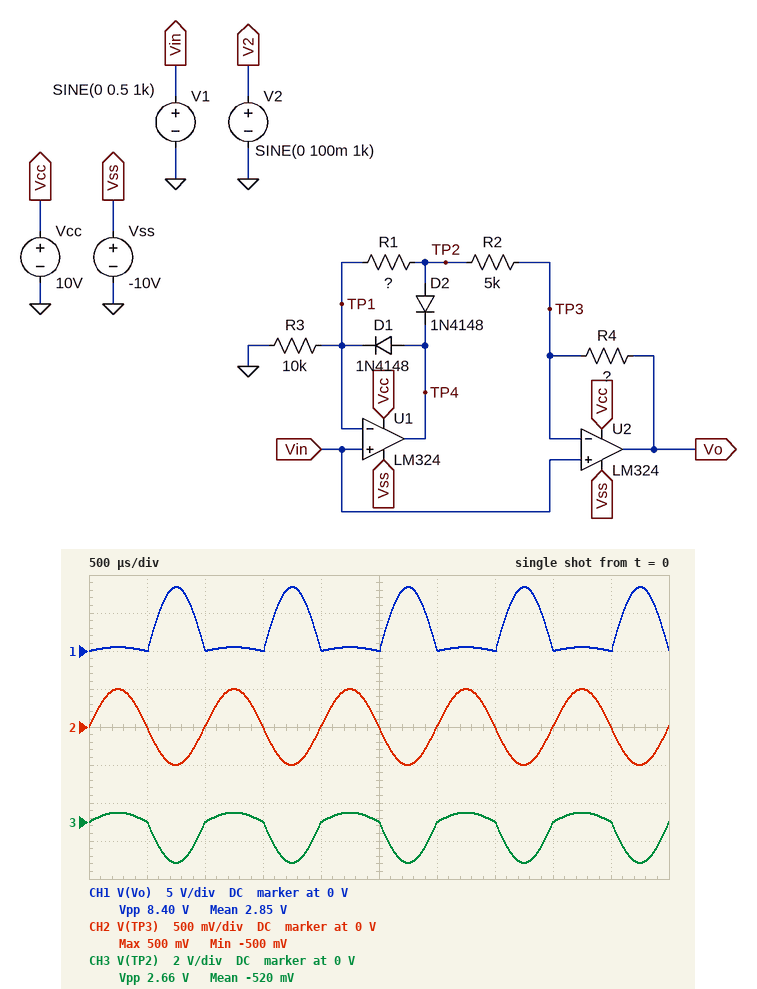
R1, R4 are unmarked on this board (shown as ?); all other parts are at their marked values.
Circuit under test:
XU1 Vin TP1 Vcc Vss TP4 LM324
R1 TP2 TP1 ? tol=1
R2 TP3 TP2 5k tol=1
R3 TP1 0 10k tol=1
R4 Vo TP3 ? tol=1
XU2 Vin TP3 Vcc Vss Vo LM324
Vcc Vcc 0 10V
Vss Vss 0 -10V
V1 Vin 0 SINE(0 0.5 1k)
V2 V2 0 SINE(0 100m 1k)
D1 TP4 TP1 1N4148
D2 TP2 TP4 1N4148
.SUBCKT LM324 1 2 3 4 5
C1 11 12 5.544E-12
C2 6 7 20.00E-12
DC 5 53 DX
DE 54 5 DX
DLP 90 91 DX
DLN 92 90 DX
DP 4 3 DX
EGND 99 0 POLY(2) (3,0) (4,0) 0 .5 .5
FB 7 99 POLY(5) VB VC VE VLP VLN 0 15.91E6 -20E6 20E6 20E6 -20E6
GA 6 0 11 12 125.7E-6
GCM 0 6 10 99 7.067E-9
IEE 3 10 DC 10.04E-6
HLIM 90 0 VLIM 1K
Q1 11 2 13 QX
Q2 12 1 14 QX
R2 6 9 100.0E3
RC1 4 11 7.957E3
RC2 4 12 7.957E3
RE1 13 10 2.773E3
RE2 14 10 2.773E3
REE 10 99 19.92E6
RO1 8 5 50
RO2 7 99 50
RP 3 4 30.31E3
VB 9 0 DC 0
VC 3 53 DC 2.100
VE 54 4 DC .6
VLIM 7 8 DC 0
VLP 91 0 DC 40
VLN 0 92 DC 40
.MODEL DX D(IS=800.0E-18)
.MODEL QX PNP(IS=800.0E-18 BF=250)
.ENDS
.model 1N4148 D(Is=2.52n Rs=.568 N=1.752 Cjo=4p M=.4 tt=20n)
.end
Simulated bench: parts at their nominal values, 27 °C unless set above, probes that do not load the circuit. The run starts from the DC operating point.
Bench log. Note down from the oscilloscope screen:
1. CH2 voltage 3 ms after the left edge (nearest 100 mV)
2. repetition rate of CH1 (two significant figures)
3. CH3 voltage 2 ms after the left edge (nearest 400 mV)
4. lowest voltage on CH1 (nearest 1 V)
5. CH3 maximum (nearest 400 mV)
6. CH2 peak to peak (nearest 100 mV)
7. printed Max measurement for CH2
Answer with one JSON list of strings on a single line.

["0 V", "1.0 kHz", "0 V", "0 V", "400 mV", "1.0 V", "500 mV"]
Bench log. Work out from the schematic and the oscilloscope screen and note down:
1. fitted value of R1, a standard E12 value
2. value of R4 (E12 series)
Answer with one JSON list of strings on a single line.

["33 kΩ", "27 kΩ"]
